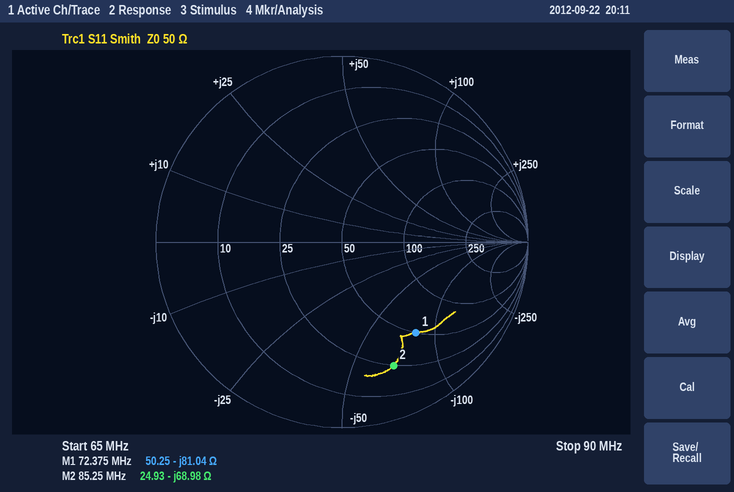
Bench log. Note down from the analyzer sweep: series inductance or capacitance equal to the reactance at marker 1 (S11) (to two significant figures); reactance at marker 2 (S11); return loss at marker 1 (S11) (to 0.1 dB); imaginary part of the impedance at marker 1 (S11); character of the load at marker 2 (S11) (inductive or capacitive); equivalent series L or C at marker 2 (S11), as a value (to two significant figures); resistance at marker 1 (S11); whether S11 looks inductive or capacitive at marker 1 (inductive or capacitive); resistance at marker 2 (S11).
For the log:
27 pF
-68.98 Ω
4.0 dB
-81.04 Ω
capacitive
27 pF
50.25 Ω
capacitive
24.93 Ω
